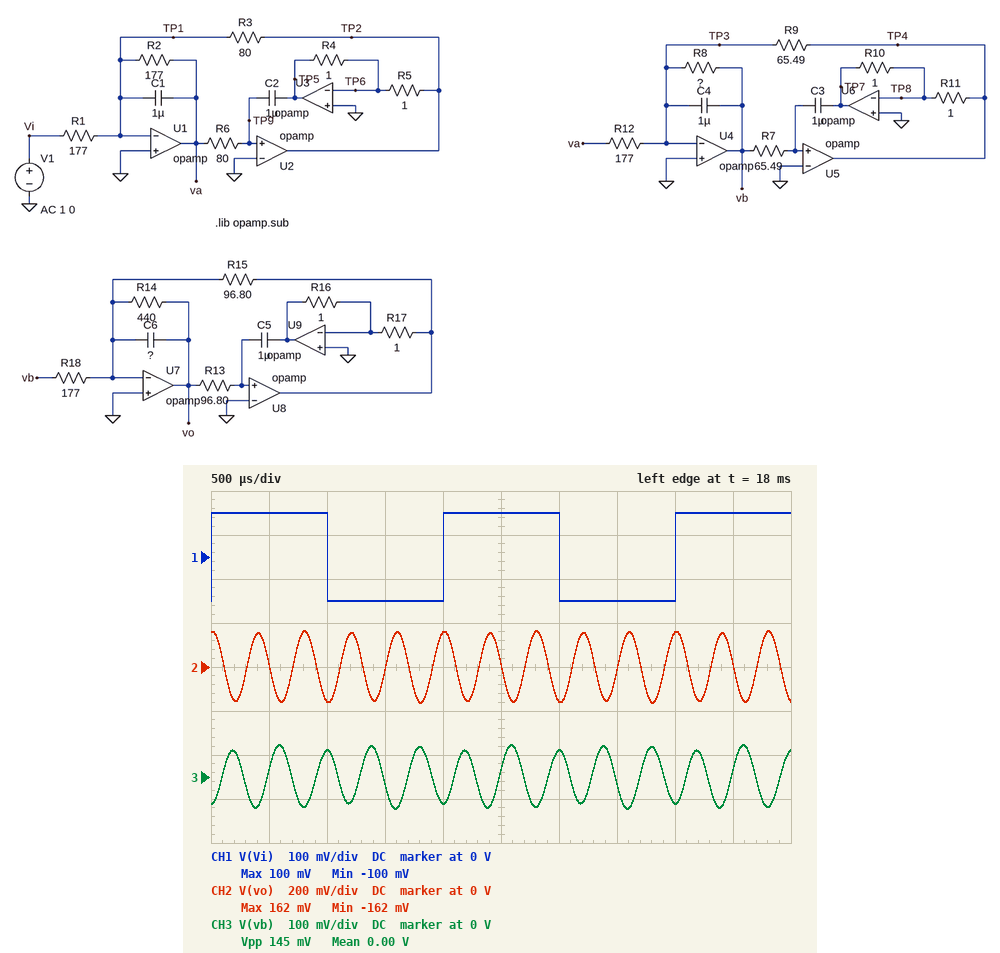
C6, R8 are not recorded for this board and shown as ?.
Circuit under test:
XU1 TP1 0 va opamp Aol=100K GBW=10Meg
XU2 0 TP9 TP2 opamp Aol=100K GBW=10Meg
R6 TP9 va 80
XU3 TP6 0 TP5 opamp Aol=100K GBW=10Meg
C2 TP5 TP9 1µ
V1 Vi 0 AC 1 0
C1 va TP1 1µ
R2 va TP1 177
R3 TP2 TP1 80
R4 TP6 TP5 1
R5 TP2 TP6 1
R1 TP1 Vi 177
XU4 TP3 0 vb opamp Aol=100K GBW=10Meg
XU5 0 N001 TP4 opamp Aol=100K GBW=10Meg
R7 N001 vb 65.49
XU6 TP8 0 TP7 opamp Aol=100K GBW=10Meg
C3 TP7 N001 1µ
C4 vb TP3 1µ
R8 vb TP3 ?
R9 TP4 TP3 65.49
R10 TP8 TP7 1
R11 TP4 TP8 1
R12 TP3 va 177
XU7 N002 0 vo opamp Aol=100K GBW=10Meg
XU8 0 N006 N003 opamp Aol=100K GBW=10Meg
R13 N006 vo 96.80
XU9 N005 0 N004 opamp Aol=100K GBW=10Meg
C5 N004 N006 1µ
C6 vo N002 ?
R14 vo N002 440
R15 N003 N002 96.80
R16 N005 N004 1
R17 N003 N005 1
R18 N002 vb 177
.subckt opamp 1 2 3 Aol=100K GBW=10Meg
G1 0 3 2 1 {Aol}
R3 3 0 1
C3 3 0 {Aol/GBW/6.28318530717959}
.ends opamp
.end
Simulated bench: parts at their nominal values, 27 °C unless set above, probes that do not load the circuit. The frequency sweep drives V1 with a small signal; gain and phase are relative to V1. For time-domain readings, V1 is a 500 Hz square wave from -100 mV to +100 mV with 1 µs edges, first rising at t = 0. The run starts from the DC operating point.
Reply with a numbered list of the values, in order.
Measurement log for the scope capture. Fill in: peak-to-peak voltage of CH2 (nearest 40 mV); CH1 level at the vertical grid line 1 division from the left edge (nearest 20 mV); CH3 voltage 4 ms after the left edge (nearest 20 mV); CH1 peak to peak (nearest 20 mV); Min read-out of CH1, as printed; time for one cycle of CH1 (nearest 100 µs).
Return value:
1. 320 mV
2. 100 mV
3. -60 mV
4. 200 mV
5. -100 mV
6. 2.0 ms
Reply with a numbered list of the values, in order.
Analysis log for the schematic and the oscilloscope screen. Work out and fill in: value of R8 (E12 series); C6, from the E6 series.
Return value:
1. 820 Ω
2. 470 nF
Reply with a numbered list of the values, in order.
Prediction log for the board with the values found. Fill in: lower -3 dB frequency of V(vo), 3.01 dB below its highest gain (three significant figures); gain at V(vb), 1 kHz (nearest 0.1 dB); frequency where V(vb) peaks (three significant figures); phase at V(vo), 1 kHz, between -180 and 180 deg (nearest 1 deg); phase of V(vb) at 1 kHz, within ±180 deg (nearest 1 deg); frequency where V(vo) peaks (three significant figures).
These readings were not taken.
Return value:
1. 2.32 kHz
2. -25.5 dB
3. 2.42 kHz
4. 62 deg
5. 161 deg
6. 2.42 kHz
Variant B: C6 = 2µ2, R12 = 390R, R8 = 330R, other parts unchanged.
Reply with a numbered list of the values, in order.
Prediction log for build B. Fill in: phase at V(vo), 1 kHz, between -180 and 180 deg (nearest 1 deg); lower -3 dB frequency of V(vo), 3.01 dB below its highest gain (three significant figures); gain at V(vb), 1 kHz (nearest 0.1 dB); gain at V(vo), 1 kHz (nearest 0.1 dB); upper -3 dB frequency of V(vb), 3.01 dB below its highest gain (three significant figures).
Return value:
1. 32 deg
2. 1.92 kHz
3. -32.4 dB
4. -29.1 dB
5. 2.59 kHz
